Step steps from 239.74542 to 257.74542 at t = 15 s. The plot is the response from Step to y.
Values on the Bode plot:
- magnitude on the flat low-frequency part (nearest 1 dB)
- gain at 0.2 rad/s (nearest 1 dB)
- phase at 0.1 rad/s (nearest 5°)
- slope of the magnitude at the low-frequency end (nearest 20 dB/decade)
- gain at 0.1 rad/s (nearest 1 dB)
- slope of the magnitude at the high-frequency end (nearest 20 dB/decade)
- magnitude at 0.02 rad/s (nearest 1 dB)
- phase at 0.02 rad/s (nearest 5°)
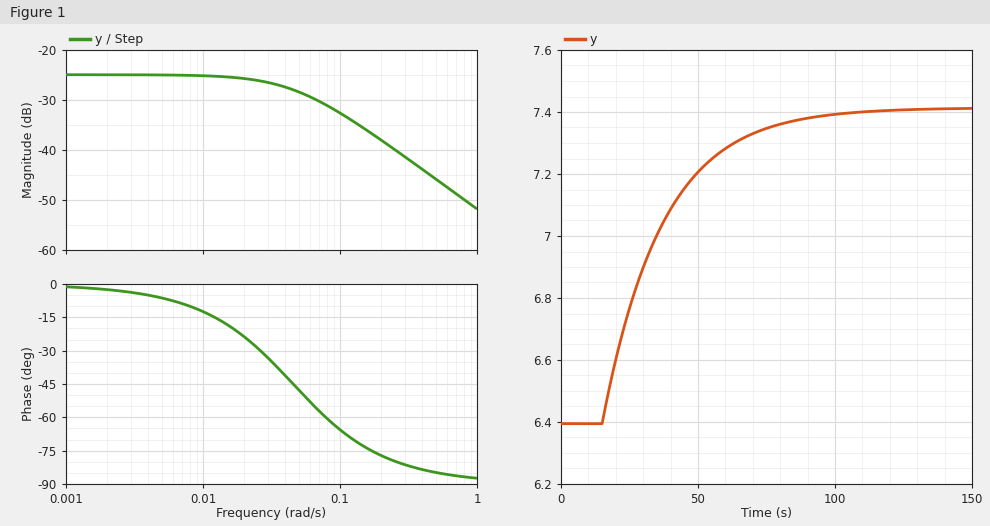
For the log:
-25 dB
-38 dB
-65°
0 dB/decade
-33 dB
-20 dB/decade
-26 dB
-25°
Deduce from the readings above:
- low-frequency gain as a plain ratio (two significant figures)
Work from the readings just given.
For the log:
0.056
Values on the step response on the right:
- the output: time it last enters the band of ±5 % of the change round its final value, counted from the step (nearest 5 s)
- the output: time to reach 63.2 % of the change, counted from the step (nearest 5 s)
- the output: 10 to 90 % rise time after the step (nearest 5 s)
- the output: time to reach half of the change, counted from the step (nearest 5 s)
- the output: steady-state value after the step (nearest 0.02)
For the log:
65 s
20 s
50 s
15 s
7.42
